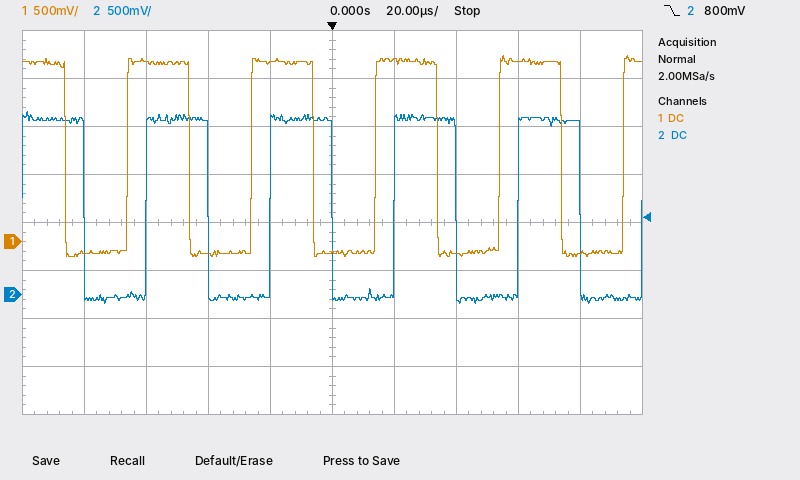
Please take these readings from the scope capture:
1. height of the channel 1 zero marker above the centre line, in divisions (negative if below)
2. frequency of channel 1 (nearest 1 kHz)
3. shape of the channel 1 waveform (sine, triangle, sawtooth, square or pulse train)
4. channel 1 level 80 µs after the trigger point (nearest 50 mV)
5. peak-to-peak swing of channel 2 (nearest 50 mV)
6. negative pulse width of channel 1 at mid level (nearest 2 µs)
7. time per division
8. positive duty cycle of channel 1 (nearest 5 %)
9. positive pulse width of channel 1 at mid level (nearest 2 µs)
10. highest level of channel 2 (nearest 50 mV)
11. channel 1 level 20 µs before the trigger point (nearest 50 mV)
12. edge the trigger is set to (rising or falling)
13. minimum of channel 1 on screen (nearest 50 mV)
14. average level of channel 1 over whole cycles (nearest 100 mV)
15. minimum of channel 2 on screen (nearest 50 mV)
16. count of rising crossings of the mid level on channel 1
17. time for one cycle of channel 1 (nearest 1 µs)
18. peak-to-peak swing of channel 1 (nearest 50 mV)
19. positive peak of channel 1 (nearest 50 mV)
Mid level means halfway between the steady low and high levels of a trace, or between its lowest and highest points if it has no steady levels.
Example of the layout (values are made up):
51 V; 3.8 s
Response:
-0.4 div; 25 kHz; square; -100 mV; 2.00 V; 20 µs; 20 µs; 50 %; 20 µs; 1.90 V; 1.85 V; falling; -150 mV; 900 mV; -100 mV; 5; 40 µs; 2.10 V; 1.95 V
